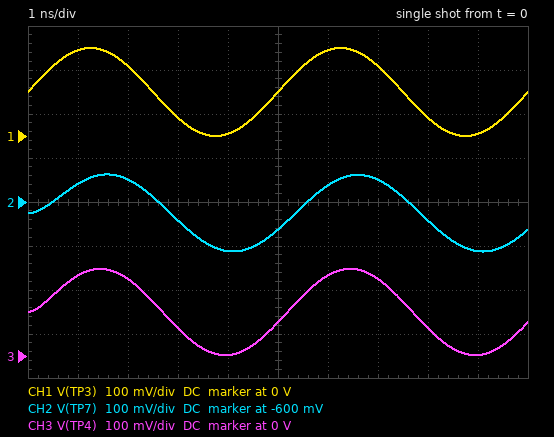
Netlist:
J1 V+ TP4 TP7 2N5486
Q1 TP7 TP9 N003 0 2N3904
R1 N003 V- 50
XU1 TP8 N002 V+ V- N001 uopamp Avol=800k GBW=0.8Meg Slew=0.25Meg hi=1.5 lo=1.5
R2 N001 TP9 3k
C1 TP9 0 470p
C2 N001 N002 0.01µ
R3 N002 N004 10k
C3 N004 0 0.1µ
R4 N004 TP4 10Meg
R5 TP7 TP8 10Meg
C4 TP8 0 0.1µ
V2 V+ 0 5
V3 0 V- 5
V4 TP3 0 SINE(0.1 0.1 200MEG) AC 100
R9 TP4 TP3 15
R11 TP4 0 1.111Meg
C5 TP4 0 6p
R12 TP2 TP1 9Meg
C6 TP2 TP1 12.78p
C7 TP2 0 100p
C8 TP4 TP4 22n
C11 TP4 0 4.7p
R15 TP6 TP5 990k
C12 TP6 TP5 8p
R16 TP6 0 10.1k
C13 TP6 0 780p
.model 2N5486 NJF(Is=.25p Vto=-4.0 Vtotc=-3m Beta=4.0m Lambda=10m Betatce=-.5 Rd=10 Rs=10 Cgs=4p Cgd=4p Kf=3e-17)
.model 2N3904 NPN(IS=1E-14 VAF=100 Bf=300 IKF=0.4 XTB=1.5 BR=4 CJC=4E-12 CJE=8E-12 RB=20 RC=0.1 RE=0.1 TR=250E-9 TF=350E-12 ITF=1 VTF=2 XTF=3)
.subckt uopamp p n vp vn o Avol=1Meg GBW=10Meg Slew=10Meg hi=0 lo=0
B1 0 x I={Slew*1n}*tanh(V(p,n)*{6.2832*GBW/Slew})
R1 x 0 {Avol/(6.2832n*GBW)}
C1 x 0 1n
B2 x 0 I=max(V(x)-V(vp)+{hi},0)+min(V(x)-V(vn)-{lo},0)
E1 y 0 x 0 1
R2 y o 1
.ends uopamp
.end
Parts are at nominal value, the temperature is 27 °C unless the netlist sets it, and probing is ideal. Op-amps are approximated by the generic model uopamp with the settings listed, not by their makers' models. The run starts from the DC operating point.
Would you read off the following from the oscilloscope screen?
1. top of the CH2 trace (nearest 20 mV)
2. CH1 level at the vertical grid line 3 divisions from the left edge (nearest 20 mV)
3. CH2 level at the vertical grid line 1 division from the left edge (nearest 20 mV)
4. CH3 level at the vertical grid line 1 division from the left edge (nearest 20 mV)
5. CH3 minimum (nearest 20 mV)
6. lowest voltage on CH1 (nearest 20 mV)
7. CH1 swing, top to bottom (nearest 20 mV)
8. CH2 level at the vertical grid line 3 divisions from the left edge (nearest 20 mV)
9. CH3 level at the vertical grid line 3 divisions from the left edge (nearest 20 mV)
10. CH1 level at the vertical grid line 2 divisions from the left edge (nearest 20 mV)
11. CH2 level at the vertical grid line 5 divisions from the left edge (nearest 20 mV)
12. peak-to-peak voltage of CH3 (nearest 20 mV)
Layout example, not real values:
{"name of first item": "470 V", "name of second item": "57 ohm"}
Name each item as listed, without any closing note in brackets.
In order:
{"top of the CH2 trace": "-540 mV", "CH1 level at the vertical grid line 3 divisions from the left edge": "40 mV", "CH2 level at the vertical grid line 1 division from the left edge": "-560 mV", "CH3 level at the vertical grid line 1 division from the left edge": "180 mV", "CH3 minimum": "0 V", "lowest voltage on CH1": "0 V", "CH1 swing, top to bottom": "200 mV", "CH2 level at the vertical grid line 3 divisions from the left edge": "-640 mV", "CH3 level at the vertical grid line 3 divisions from the left edge": "60 mV", "CH1 level at the vertical grid line 2 divisions from the left edge": "160 mV", "CH2 level at the vertical grid line 5 divisions from the left edge": "-660 mV", "peak-to-peak voltage of CH3": "200 mV"}
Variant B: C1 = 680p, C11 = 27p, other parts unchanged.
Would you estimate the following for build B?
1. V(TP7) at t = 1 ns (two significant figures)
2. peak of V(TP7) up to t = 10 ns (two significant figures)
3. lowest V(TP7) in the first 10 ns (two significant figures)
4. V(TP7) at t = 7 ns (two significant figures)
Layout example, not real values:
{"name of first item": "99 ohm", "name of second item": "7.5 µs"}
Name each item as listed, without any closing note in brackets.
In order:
{"V(TP7) at t = 1 ns": "-580 mV", "peak of V(TP7) up to t = 10 ns": "-550 mV", "lowest V(TP7) in the first 10 ns": "-700 mV", "V(TP7) at t = 7 ns": "-550 mV"}
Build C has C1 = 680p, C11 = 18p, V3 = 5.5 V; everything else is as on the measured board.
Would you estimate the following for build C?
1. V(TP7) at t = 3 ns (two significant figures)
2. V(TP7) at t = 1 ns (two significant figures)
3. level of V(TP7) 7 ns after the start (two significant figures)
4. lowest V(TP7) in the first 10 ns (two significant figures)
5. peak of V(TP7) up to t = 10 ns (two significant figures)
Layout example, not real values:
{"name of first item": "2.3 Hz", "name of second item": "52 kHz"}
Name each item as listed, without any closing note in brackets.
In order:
{"V(TP7) at t = 3 ns": "-920 mV", "V(TP7) at t = 1 ns": "-870 mV", "level of V(TP7) 7 ns after the start": "-850 mV", "lowest V(TP7) in the first 10 ns": "-1.0 V", "peak of V(TP7) up to t = 10 ns": "-840 mV"}
